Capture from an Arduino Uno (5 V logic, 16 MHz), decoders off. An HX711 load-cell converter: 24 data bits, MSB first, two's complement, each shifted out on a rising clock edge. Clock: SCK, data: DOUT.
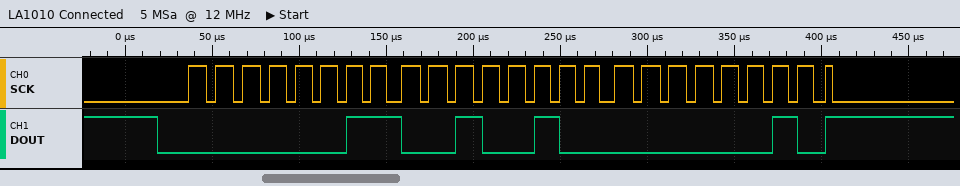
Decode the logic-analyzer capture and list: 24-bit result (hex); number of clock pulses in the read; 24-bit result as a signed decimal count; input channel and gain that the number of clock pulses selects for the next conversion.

0x032402
25
205826
channel A, gain 128
